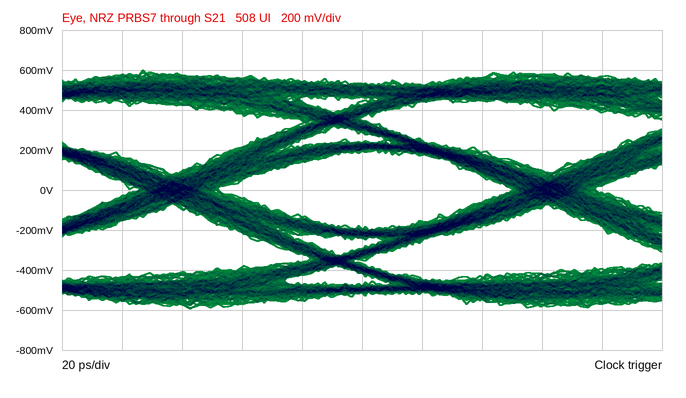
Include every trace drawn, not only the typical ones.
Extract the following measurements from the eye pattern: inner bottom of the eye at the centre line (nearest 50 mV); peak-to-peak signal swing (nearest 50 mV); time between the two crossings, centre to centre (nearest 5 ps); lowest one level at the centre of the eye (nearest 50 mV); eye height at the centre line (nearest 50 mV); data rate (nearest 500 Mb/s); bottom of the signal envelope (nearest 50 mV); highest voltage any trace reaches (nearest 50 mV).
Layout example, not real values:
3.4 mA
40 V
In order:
-200 mV
1.20 V
125 ps
200 mV
400 mV
8.0 Gb/s
-600 mV
600 mV
